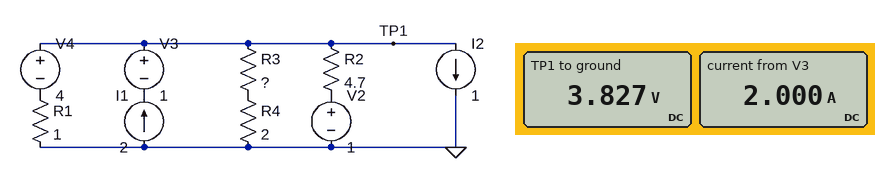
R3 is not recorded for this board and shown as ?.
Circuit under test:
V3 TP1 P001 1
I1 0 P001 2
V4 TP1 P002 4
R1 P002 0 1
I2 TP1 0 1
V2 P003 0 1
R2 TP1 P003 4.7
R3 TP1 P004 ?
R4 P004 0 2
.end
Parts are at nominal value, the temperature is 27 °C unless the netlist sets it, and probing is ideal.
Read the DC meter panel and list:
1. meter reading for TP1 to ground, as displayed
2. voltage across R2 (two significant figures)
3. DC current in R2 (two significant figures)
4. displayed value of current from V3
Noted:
3.827 V
2.8 V
600 mA
2.000 A
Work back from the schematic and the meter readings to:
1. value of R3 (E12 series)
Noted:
4.7 Ω
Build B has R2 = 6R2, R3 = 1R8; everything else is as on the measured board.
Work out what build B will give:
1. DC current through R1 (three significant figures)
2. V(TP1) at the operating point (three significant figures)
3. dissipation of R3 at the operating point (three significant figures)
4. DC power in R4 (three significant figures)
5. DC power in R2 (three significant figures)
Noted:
377 mA
3.62 V
1.64 W
1.82 W
1.11 W
